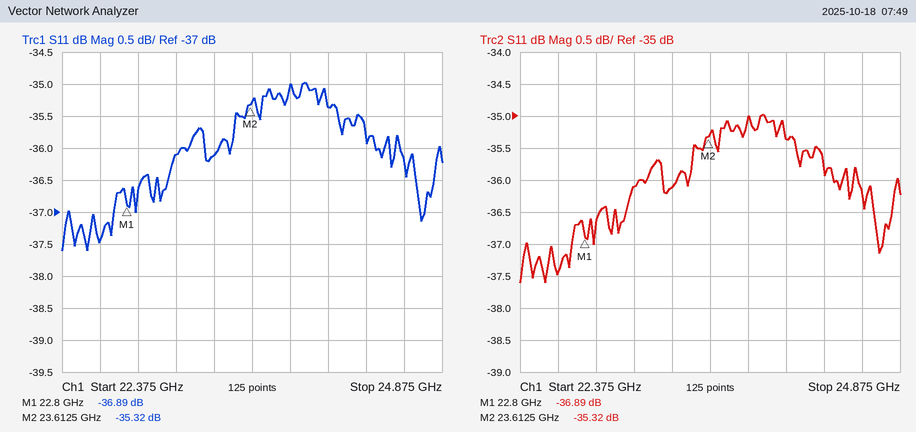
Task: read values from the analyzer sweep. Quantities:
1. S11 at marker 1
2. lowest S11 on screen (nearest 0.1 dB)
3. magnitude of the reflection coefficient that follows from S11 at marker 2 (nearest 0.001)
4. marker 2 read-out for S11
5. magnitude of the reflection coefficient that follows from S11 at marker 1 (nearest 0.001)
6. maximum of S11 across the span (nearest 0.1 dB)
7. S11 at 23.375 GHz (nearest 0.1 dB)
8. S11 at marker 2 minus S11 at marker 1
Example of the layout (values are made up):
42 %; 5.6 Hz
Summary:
-36.89 dB; -37.6 dB; 0.017; -35.32 dB; 0.014; -35.0 dB; -36.1 dB; 1.57 dB
